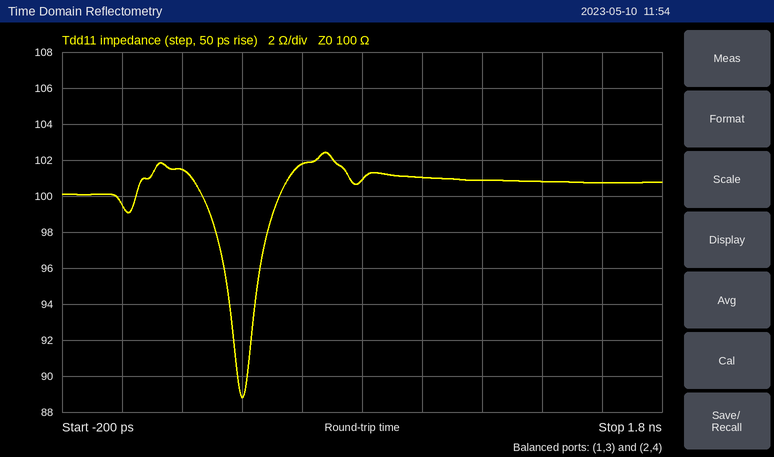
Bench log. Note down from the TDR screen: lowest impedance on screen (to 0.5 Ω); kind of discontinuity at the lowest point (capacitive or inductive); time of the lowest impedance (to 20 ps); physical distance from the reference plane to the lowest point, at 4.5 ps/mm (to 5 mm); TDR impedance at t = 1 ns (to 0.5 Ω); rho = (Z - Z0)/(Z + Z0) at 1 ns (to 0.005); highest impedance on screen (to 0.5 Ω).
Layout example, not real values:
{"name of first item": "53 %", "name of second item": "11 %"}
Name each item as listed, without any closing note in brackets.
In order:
{"lowest impedance on screen": "89.0 Ω", "kind of discontinuity at the lowest point": "capacitive", "time of the lowest impedance": "400 ps", "physical distance from the reference plane to the lowest point, at 4.5 ps/mm": "45 mm", "TDR impedance at t = 1 ns": "101.0 Ω", "rho = (Z - Z0)/(Z + Z0) at 1 ns": "+0.005", "highest impedance on screen": "102.5 Ω"}
